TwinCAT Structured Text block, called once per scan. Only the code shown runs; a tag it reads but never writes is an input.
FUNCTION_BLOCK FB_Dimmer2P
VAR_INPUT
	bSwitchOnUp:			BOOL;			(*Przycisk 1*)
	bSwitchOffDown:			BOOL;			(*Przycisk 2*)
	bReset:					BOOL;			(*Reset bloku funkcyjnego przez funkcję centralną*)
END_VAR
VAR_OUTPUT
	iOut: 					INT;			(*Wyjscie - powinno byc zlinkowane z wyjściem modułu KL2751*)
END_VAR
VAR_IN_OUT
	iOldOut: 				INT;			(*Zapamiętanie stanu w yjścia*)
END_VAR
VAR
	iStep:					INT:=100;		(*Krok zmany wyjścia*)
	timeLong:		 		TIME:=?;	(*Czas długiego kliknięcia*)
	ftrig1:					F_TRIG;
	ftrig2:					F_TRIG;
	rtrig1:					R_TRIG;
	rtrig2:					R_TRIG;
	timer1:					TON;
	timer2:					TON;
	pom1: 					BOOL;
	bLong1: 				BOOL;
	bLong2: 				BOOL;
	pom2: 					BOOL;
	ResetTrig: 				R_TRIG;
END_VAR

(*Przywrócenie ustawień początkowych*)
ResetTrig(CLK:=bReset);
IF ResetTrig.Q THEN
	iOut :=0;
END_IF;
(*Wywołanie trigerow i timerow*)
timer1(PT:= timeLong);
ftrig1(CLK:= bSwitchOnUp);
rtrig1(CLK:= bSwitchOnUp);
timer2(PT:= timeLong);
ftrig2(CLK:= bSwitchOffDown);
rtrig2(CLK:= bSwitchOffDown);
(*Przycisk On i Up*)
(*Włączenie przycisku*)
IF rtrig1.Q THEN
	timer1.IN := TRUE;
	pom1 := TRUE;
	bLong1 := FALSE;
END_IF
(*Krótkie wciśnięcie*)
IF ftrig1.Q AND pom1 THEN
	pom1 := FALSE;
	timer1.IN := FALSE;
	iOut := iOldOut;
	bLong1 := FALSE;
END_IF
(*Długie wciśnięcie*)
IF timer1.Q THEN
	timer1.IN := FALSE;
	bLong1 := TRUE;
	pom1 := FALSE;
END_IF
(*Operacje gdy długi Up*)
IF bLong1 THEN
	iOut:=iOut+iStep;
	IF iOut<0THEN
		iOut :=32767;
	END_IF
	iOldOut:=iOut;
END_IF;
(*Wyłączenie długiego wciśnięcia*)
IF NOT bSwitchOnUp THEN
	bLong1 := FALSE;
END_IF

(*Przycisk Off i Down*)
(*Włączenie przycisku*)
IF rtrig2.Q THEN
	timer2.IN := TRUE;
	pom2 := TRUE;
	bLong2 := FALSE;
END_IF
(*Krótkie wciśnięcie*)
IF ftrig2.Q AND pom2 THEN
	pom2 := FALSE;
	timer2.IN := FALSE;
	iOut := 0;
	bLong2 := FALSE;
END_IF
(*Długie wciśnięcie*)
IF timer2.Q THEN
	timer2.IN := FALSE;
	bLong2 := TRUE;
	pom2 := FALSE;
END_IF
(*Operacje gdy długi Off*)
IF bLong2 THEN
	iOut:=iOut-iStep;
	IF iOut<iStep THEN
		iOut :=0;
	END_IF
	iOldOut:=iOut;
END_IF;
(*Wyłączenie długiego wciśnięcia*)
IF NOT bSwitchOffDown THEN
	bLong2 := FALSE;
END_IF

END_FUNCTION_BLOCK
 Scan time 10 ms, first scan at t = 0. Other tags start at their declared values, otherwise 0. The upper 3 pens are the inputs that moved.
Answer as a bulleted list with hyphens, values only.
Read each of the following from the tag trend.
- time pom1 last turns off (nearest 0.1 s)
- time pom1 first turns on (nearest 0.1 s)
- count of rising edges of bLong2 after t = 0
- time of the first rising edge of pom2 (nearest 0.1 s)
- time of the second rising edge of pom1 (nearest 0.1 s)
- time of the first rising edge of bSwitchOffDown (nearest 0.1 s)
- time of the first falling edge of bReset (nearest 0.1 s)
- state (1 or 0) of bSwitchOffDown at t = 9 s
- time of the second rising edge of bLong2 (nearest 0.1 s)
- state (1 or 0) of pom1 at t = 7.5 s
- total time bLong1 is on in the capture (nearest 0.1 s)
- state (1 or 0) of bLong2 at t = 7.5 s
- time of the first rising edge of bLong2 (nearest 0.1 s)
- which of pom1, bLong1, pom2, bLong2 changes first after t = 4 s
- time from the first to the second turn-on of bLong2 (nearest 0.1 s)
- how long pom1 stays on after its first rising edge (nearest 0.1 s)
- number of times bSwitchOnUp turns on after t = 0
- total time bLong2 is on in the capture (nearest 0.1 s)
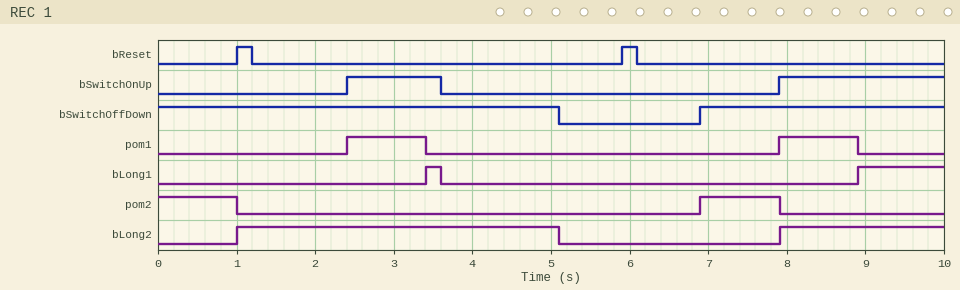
- 8.9 s
- 2.4 s
- 2
- 6.9 s
- 7.9 s
- 6.9 s
- 1.2 s
- 1
- 7.9 s
- 0
- 1.3 s
- 0
- 1.0 s
- bLong2
- 6.9 s
- 1.0 s
- 2
- 6.2 s
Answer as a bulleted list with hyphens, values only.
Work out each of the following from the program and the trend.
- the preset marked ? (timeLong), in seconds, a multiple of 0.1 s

- 1.0 s
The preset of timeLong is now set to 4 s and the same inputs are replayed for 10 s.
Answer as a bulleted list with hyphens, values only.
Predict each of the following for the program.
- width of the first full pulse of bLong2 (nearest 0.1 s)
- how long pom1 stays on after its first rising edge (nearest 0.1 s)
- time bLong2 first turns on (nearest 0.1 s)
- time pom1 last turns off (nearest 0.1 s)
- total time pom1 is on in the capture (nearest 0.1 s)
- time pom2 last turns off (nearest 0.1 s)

- 1.1 s
- 1.2 s
- 4.0 s
- 3.6 s
- 3.3 s
- 4.0 s
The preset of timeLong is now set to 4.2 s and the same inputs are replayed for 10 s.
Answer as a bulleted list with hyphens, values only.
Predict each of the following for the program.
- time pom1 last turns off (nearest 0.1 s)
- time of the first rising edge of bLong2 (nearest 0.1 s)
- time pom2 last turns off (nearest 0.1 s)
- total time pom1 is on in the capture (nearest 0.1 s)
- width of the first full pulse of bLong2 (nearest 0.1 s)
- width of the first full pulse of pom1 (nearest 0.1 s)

- 3.6 s
- 4.2 s
- 4.2 s
- 3.3 s
- 0.9 s
- 1.2 s
